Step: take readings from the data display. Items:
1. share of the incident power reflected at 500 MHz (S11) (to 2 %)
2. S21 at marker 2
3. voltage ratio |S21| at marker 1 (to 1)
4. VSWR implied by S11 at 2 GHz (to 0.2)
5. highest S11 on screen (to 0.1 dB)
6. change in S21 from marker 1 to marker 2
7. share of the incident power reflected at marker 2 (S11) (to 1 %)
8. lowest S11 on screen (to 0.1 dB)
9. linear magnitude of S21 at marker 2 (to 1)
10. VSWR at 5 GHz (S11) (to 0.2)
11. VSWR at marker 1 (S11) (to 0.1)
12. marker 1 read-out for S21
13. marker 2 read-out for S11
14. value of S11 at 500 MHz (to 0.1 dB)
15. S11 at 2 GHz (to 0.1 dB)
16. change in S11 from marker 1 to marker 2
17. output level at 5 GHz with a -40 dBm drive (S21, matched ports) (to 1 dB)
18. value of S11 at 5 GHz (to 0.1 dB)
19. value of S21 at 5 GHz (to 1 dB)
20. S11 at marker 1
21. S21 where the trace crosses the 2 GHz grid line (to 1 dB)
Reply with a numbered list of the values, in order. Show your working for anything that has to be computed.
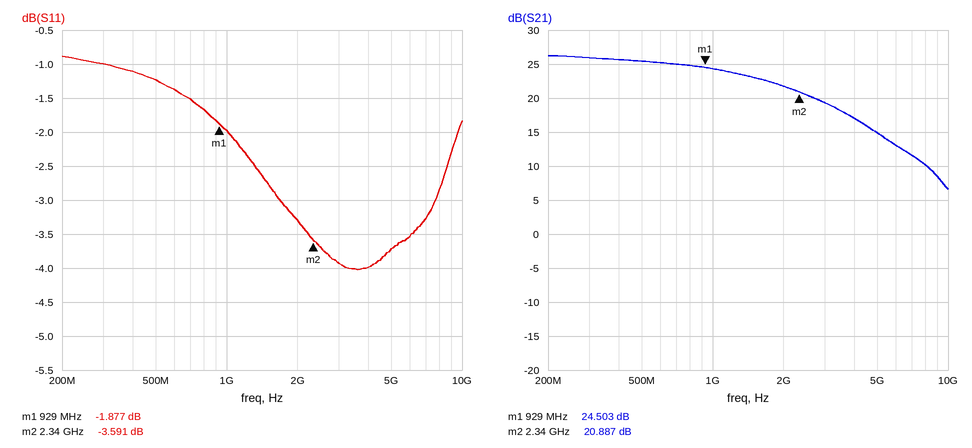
1. 10^(-1.2/10) ≈ 76 %
2. 20.887 dB
3. 10^(24.503/20) ≈ 17
4. |Γ| = 10^(-3.3/20) = 0.6839; VSWR = (1 + 0.6839)/(1 − 0.6839) ≈ 5.33, so 5.4 to the nearest 0.2
5. -0.9 dB
6. 20.887 − (24.503) = -3.616 dB
7. 10^(-3.591/10) ≈ 44 %
8. -4.0 dB
9. 10^(20.887/20) ≈ 11
10. |Γ| = 10^(-3.7/20) = 0.6531; VSWR = (1 + 0.6531)/(1 − 0.6531) ≈ 4.8
11. (1 + 0.8057)/(1 − 0.8057) ≈ 9.3
12. 24.503 dB
13. -3.591 dB
14. -1.2 dB
15. -3.3 dB
16. -3.591 − (-1.877) = -1.714 dB
17. -40 dBm + (15 dB) = -25 dBm
18. -3.7 dB
19. 15 dB
20. -1.877 dB
21. 22 dB
